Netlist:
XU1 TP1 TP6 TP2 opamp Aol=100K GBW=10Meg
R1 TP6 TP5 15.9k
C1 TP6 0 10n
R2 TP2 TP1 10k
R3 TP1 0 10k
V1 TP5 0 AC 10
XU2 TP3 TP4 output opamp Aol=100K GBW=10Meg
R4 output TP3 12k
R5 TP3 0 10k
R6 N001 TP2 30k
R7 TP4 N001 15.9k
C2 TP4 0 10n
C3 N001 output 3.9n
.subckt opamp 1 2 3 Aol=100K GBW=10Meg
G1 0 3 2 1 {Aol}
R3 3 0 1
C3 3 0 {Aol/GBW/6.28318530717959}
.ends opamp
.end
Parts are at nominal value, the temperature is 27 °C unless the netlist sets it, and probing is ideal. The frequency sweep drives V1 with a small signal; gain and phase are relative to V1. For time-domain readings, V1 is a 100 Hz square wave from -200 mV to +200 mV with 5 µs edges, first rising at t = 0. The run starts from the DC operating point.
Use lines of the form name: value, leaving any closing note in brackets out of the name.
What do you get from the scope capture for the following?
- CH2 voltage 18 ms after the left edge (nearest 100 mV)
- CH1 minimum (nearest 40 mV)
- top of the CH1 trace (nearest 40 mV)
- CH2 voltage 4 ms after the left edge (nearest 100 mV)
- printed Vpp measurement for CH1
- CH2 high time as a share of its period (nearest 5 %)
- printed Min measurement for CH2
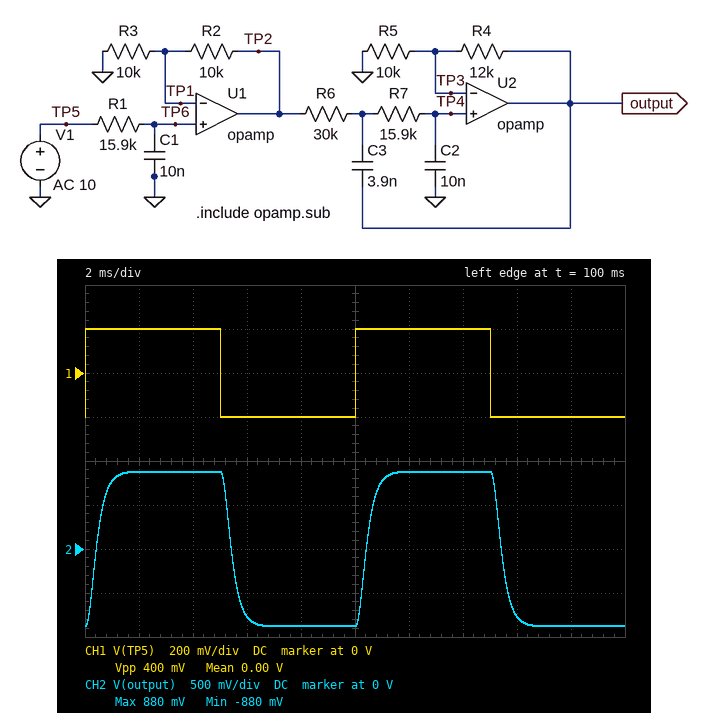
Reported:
CH2 voltage 18 ms after the left edge: -900 mV
CH1 minimum: -200 mV
top of the CH1 trace: 200 mV
CH2 voltage 4 ms after the left edge: 900 mV
printed Vpp measurement for CH1: 400 mV
CH2 high time as a share of its period: 50 %
printed Min measurement for CH2: -880 mV
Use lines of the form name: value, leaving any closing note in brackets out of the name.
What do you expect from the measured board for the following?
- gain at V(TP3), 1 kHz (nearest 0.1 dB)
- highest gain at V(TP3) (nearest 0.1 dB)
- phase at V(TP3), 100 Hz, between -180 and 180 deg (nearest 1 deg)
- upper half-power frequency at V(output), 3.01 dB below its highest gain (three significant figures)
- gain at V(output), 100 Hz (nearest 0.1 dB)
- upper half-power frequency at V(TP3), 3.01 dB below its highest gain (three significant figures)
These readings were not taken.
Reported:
gain at V(TP3), 1 kHz: -3.1 dB
highest gain at V(TP3): 6.0 dB
phase at V(TP3), 100 Hz, between -180 and 180 deg: -17 deg
upper half-power frequency at V(output), 3.01 dB below its highest gain: 483 Hz
gain at V(output), 100 Hz: 12.7 dB
upper half-power frequency at V(TP3), 3.01 dB below its highest gain: 483 Hz
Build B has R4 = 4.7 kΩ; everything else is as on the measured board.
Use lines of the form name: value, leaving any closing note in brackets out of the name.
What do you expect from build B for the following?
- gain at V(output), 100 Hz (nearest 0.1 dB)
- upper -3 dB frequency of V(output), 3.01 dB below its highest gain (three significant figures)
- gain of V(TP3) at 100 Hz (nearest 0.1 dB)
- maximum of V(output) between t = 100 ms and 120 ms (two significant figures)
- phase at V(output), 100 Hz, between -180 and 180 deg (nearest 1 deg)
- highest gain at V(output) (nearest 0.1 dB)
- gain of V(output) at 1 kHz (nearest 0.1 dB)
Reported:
gain at V(output), 100 Hz: 9.1 dB
upper -3 dB frequency of V(output), 3.01 dB below its highest gain: 384 Hz
gain of V(TP3) at 100 Hz: 5.8 dB
maximum of V(output) between t = 100 ms and 120 ms: 590 mV
phase at V(output), 100 Hz, between -180 and 180 deg: -20 deg
highest gain at V(output): 9.4 dB
gain of V(output) at 1 kHz: -1.8 dB
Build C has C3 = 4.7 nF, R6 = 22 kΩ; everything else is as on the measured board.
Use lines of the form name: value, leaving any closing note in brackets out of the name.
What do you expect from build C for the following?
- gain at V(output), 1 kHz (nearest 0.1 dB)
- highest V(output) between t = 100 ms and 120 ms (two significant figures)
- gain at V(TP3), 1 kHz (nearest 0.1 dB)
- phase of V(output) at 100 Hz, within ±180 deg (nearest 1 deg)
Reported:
gain at V(output), 1 kHz: 5.6 dB
highest V(output) between t = 100 ms and 120 ms: 880 mV
gain at V(TP3), 1 kHz: -1.3 dB
phase of V(output) at 100 Hz, within ±180 deg: -15 deg
